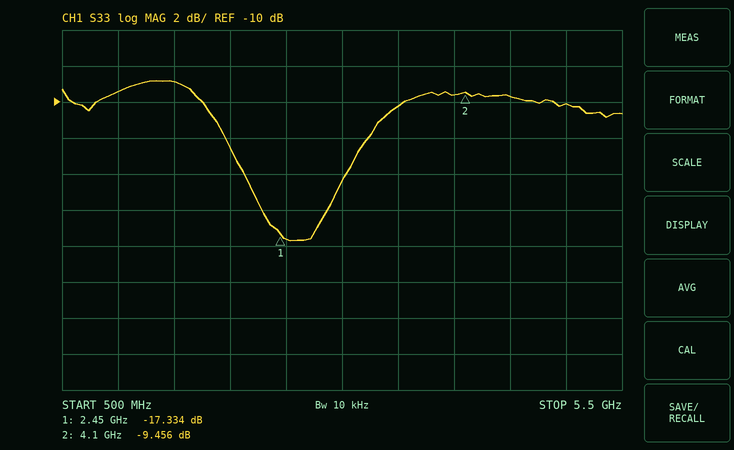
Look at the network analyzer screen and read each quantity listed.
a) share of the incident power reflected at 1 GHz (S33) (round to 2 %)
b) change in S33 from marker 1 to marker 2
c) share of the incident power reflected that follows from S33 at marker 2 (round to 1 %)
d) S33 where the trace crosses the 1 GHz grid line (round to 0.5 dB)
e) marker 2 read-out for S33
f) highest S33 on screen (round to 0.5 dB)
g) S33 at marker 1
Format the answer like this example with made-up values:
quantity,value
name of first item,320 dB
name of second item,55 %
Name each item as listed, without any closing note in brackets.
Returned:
quantity,value
share of the incident power reflected at 1 GHz (S33),12 %
change in S33 from marker 1 to marker 2,7.878 dB
share of the incident power reflected that follows from S33 at marker 2,11 %
S33 where the trace crosses the 1 GHz grid line,-9.5 dB
marker 2 read-out for S33,-9.456 dB
highest S33 on screen,-9.0 dB
S33 at marker 1,-17.334 dB
